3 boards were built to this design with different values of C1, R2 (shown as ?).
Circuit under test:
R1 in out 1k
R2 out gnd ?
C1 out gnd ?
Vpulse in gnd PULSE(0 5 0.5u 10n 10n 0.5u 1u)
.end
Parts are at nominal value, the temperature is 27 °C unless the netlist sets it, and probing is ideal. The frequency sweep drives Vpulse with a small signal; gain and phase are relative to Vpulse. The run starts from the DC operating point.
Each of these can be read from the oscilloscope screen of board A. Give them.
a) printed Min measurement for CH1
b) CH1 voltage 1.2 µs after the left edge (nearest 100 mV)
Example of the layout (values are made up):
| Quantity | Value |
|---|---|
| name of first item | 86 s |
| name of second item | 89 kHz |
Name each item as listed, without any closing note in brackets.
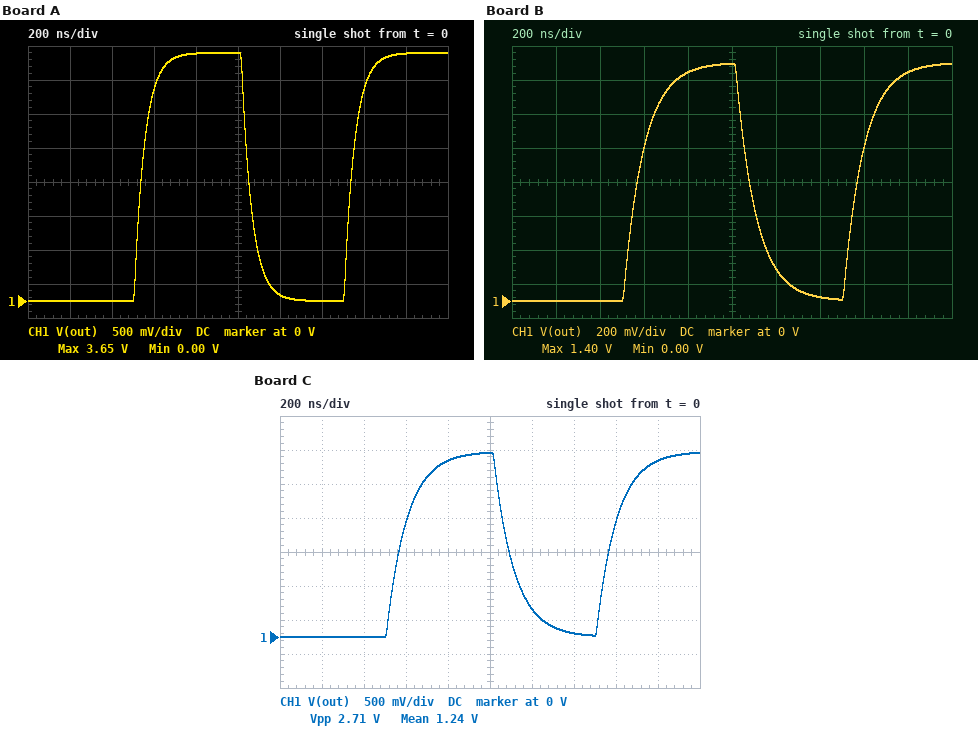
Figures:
| Quantity | Value |
|---|---|
| printed Min measurement for CH1 | 0.00 V |
| CH1 voltage 1.2 µs after the left edge | 100 mV |
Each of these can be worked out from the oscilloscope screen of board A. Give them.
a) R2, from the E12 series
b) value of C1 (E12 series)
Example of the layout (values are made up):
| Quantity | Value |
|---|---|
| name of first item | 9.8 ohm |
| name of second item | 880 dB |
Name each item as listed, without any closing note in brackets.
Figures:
| Quantity | Value |
|---|---|
| R2, from the E12 series | 2.7 kΩ |
| value of C1 | 68 pF |
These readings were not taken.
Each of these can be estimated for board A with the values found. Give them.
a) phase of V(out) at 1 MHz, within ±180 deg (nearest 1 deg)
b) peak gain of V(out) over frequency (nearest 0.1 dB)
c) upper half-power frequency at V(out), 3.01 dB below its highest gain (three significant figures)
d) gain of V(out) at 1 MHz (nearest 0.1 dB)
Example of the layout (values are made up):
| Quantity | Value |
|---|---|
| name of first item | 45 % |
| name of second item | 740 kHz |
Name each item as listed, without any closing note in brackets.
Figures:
| Quantity | Value |
|---|---|
| phase of V(out) at 1 MHz, within ±180 deg | -17 deg |
| peak gain of V(out) over frequency | -2.7 dB |
| upper half-power frequency at V(out), 3.01 dB below its highest gain | 3.21 MHz |
| gain of V(out) at 1 MHz | -3.1 dB |
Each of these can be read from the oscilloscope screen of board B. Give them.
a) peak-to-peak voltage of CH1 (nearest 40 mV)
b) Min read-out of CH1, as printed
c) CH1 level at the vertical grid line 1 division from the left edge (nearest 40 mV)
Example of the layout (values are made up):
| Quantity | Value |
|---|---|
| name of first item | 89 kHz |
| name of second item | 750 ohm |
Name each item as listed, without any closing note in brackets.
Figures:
| Quantity | Value |
|---|---|
| peak-to-peak voltage of CH1 | 1.40 V |
| Min read-out of CH1, as printed | 0.00 V |
| CH1 level at the vertical grid line 1 division from the left edge | 0 V |
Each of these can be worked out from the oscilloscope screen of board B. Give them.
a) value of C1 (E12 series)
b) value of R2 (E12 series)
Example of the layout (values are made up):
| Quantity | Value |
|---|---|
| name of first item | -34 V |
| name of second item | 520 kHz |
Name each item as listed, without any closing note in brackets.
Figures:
| Quantity | Value |
|---|---|
| value of C1 | 330 pF |
| value of R2 | 390 Ω |
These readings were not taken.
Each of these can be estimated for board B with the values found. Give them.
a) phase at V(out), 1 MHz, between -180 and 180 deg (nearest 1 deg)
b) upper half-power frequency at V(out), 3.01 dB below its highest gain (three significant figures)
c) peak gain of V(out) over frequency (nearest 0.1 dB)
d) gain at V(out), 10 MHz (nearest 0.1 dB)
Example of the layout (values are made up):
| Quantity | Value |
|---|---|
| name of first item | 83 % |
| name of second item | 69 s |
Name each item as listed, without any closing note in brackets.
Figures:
| Quantity | Value |
|---|---|
| phase at V(out), 1 MHz, between -180 and 180 deg | -30 deg |
| upper half-power frequency at V(out), 3.01 dB below its highest gain | 1.72 MHz |
| peak gain of V(out) over frequency | -11.0 dB |
| gain at V(out), 10 MHz | -26.5 dB |
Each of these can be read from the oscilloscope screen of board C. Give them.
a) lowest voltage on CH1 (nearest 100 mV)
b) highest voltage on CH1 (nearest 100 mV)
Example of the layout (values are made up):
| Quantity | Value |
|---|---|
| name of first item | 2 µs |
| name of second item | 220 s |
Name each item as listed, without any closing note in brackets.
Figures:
| Quantity | Value |
|---|---|
| lowest voltage on CH1 | 0 V |
| highest voltage on CH1 | 2.7 V |
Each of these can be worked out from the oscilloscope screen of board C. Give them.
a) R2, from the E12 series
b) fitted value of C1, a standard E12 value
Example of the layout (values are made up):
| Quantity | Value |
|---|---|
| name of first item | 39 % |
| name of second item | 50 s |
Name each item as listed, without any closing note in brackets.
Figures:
| Quantity | Value |
|---|---|
| R2, from the E12 series | 1.2 kΩ |
| fitted value of C1, a standard E12 value | 180 pF |
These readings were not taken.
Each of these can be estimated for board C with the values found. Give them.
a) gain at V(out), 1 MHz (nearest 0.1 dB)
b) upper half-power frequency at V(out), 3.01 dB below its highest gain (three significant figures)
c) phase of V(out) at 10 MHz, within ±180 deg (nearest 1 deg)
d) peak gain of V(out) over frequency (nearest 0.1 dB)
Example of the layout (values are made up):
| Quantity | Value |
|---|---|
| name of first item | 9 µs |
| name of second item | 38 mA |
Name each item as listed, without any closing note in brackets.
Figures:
| Quantity | Value |
|---|---|
| gain at V(out), 1 MHz | -6.7 dB |
| upper half-power frequency at V(out), 3.01 dB below its highest gain | 1.62 MHz |
| phase of V(out) at 10 MHz, within ±180 deg | -81 deg |
| peak gain of V(out) over frequency | -5.3 dB |
